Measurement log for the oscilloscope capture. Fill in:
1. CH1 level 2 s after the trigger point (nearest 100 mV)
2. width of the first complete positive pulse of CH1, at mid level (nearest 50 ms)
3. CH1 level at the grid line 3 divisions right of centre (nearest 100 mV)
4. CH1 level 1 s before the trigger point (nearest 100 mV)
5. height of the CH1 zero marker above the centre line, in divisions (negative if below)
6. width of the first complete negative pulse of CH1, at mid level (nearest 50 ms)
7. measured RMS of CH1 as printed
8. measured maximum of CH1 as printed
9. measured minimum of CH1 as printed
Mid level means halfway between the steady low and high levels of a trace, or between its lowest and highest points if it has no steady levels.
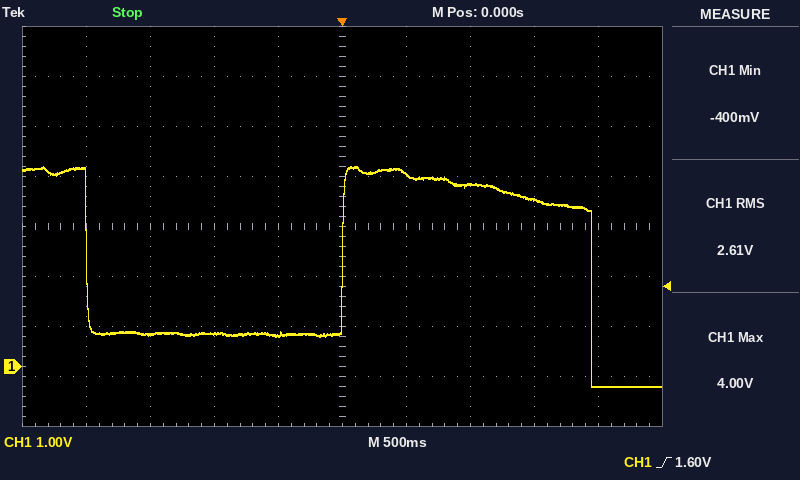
-400 mV
1.95 s
3.3 V
700 mV
-2.8 div
2.00 s
2.61 V
4.00 V
-400 mV
